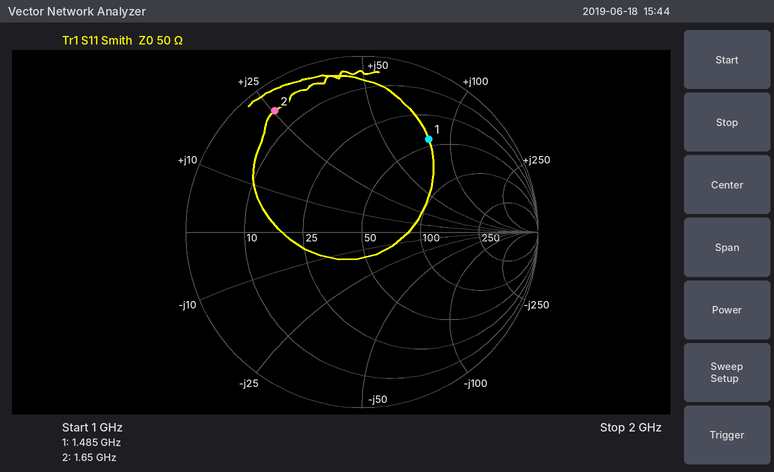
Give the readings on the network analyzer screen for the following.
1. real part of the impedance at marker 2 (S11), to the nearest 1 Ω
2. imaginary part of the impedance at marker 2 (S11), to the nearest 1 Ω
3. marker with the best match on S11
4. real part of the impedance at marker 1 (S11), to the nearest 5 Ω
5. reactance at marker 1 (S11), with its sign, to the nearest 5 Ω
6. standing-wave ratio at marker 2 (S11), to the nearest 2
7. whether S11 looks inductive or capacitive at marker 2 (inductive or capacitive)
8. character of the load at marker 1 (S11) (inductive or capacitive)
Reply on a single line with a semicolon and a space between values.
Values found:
5 Ω; +25 Ω; marker 1; 45 Ω; +80 Ω; 12; inductive; inductive
